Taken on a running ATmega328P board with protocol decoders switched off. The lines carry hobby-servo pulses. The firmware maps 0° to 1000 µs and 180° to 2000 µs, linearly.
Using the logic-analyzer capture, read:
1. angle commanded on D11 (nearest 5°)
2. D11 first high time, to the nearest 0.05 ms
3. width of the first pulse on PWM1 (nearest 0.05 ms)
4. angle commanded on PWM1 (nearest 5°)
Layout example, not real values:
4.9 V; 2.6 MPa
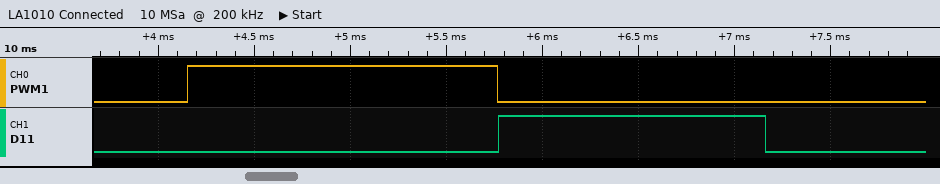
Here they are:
70°; 1.40 ms; 1.60 ms; 110°
